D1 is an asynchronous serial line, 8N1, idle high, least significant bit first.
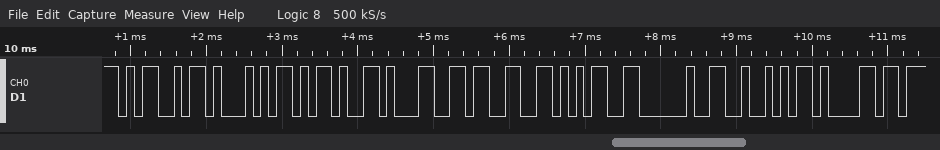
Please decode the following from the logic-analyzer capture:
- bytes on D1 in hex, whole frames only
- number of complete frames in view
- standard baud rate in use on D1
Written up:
0x4D 0x51 0x2D 0x31 0x33 0x35 0x20 0x52 0x61
9
9600 baud
